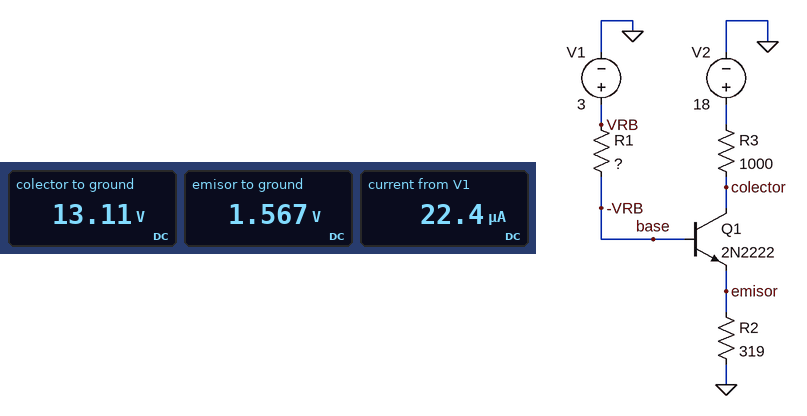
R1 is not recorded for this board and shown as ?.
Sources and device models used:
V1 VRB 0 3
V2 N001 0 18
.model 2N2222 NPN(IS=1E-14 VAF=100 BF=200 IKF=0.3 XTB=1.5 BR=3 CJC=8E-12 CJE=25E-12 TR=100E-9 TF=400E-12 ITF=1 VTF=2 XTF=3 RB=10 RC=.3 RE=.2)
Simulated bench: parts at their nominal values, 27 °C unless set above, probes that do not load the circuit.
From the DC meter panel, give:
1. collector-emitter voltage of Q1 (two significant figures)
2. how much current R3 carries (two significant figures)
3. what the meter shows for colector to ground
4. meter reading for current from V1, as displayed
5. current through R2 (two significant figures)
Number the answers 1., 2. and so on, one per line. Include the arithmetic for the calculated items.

1. 13.11 V - 1.567 V = 12 V
2. (18 V - 13.11 V) / 1 kΩ = 4.9 mA
3. 13.11 V
4. 22.4 µA
5. (1.567 V) / 319 Ω = 4.9 mA
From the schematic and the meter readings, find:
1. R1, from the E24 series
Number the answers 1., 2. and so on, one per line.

1. 33 kΩ
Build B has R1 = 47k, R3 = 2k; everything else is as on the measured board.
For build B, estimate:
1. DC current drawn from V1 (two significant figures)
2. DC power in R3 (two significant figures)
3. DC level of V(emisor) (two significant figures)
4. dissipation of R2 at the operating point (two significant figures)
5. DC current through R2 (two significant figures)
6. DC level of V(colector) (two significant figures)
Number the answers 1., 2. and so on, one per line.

1. 20 µA
2. 36 mW
3. 1.4 V
4. 5.8 mW
5. 4.3 mA
6. 9.5 V
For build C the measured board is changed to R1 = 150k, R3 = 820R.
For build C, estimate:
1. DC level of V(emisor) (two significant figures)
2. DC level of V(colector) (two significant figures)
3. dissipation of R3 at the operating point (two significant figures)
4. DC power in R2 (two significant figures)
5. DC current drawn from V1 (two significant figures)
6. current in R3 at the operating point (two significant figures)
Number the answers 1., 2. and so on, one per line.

1. 760 mV
2. 16 V
3. 4.6 mW
4. 1.8 mW
5. 10 µA
6. 2.4 mA
